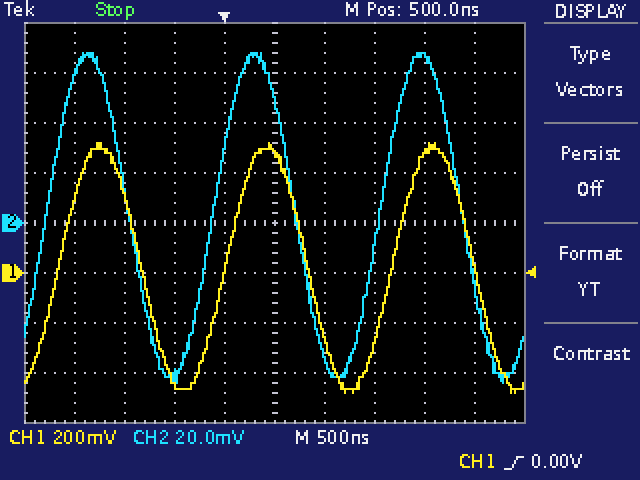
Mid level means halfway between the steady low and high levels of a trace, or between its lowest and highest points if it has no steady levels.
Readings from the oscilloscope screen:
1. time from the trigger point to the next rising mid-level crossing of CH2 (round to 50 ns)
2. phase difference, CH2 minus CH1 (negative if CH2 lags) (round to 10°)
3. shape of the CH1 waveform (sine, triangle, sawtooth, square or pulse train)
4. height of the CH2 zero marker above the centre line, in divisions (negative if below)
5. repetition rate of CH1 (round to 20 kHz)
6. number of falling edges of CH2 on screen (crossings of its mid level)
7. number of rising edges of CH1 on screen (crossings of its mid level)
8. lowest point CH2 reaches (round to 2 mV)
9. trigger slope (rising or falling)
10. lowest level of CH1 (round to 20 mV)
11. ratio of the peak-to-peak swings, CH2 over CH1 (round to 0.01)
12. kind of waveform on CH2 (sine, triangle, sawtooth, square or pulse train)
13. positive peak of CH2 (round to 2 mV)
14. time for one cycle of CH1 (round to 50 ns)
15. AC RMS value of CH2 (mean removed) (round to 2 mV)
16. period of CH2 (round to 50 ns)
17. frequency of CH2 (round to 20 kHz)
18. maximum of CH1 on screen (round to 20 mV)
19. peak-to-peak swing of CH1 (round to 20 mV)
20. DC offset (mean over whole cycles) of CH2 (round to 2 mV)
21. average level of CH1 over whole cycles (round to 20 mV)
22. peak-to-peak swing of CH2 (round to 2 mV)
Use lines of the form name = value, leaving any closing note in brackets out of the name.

time from the trigger point to the next rising mid-level crossing of CH2 = 1.55 µs
phase difference, CH2 minus CH1 (negative if CH2 lags) = +30°
shape of the CH1 waveform = sine
height of the CH2 zero marker above the centre line, in divisions = 0.0 div
repetition rate of CH1 = 600 kHz
number of falling edges of CH2 on screen = 3
number of rising edges of CH1 on screen = 3
lowest point CH2 reaches = -64 mV
trigger slope = rising
lowest level of CH1 = -480 mV
ratio of the peak-to-peak swings, CH2 over CH1 = 0.13
kind of waveform on CH2 = sine
positive peak of CH2 = 68 mV
time for one cycle of CH1 = 1.65 µs
AC RMS value of CH2 (mean removed) = 46 mV
period of CH2 = 1.65 µs
frequency of CH2 = 600 kHz
maximum of CH1 on screen = 520 mV
peak-to-peak swing of CH1 = 1.00 V
DC offset (mean over whole cycles) of CH2 = 2 mV
average level of CH1 over whole cycles = 20 mV
peak-to-peak swing of CH2 = 132 mV
